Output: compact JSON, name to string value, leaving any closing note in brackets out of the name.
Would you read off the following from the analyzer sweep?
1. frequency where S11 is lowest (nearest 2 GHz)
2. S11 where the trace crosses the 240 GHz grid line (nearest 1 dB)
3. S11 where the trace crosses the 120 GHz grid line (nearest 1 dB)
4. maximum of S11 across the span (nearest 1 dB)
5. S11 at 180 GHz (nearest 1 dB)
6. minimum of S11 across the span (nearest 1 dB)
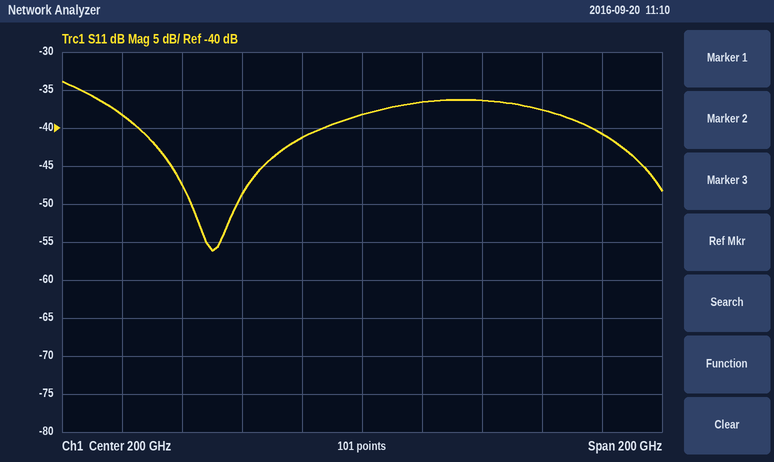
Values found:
{"frequency where S11 is lowest": "150 GHz", "S11 where the trace crosses the 240 GHz grid line": "-36 dB", "S11 where the trace crosses the 120 GHz grid line": "-38 dB", "maximum of S11 across the span": "-34 dB", "S11 at 180 GHz": "-41 dB", "minimum of S11 across the span": "-56 dB"}
